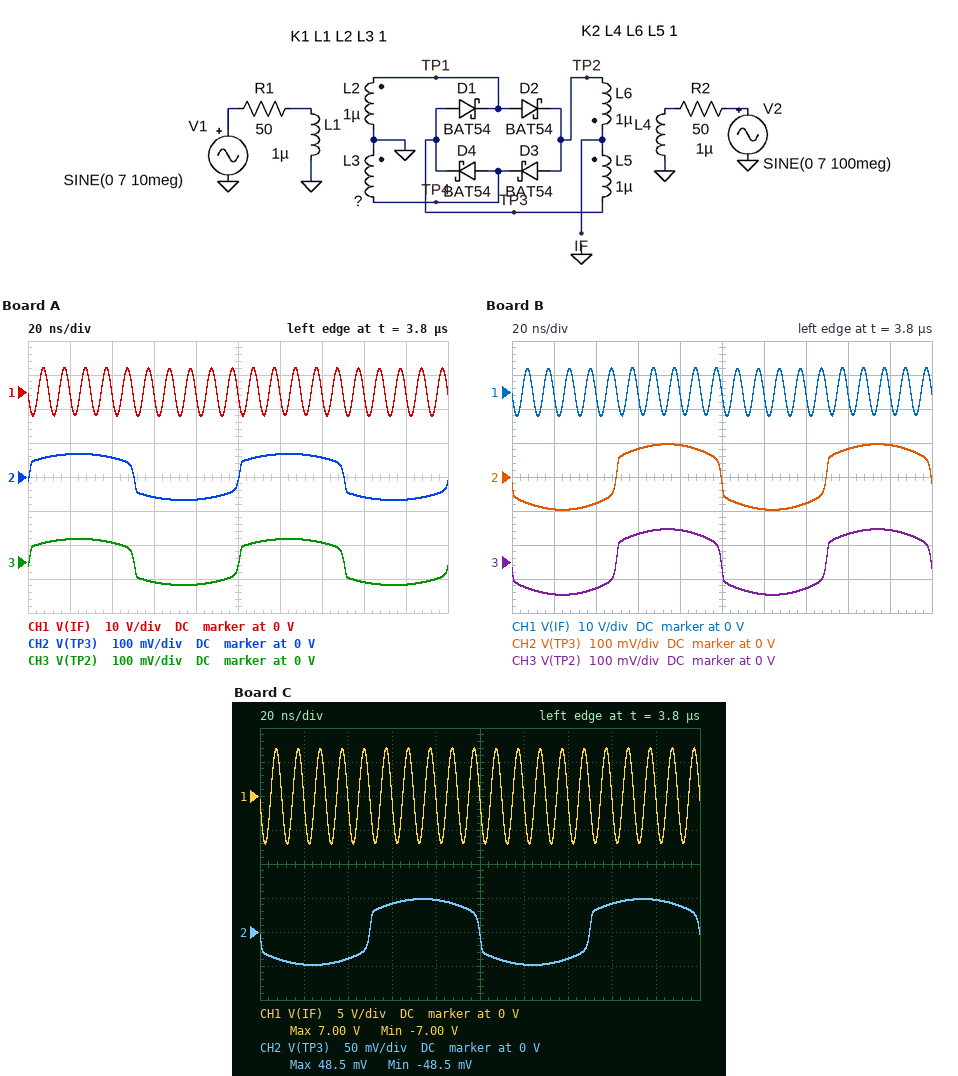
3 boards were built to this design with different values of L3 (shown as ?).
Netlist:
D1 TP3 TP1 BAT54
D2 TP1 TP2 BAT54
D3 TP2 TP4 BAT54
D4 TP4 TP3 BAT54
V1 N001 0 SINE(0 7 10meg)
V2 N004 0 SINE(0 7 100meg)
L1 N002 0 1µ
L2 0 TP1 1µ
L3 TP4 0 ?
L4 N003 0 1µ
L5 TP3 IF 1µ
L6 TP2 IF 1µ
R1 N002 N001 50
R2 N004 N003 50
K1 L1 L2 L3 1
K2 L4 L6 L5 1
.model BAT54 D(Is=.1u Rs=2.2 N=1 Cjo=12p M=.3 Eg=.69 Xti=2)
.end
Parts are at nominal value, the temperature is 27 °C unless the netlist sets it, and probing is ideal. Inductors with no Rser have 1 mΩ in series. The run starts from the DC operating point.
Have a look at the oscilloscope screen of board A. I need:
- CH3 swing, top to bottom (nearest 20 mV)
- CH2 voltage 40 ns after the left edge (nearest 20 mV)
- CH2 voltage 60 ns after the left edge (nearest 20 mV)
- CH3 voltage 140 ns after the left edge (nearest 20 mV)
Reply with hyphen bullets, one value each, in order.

- 140 mV
- 60 mV
- -60 mV
- 60 mV
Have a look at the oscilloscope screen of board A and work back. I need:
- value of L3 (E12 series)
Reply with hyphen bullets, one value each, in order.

- 1.8 µH
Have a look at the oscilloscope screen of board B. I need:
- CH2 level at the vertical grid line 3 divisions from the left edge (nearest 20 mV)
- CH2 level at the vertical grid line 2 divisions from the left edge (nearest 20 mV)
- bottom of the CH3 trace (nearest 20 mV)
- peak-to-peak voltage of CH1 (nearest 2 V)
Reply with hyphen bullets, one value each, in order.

- 80 mV
- -80 mV
- -100 mV
- 14 V
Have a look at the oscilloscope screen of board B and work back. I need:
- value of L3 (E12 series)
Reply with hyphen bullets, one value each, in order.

- 470 nH
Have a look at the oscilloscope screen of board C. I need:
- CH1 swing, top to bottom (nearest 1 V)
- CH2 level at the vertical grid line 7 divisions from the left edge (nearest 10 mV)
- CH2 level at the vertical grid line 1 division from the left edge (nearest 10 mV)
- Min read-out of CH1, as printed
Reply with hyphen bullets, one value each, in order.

- 14 V
- -40 mV
- -50 mV
- -7.00 V
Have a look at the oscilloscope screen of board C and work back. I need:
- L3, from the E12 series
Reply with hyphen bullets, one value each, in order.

- 680 nH
